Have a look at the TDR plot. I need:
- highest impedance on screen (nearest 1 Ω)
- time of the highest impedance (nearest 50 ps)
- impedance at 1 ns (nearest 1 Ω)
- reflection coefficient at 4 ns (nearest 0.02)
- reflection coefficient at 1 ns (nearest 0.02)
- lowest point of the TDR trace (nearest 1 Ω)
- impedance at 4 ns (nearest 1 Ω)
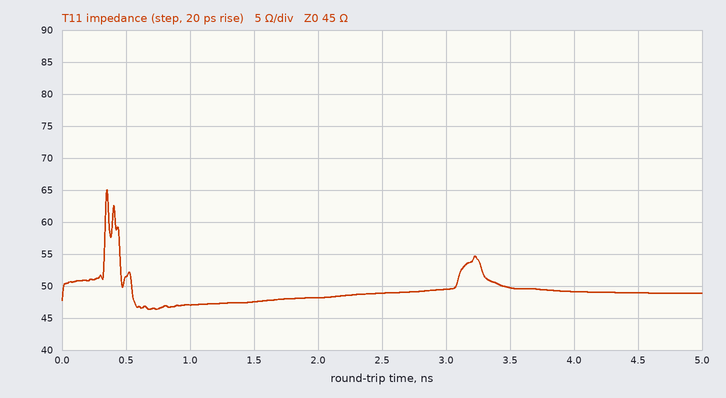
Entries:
65 Ω
350 ps
47 Ω
+0.04
+0.02
46 Ω
49 Ω
